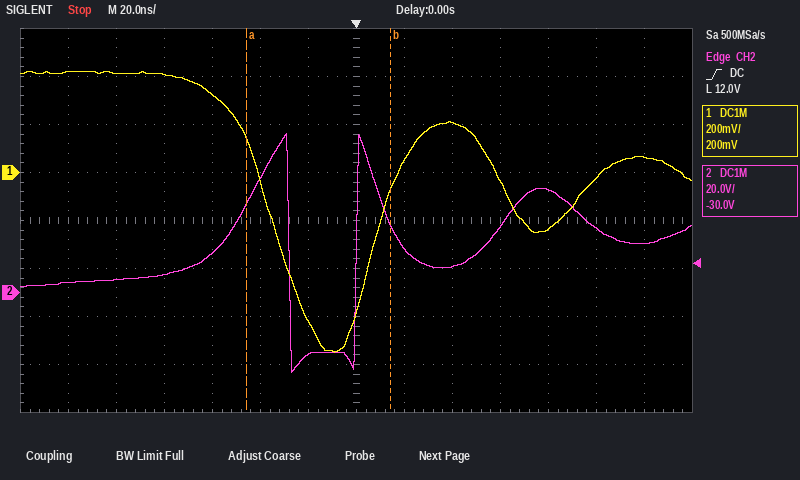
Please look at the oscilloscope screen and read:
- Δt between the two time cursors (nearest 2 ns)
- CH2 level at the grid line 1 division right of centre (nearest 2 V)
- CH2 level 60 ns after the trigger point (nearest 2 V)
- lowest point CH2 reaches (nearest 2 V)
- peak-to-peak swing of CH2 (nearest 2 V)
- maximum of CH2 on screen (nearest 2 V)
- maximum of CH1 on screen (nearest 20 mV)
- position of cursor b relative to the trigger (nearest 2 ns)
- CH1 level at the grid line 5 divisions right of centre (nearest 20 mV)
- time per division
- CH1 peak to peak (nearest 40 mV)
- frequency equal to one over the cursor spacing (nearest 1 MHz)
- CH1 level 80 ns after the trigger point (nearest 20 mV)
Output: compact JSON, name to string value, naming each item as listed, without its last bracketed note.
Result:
{"Δt between the two time cursors": "60 ns", "CH2 level at the grid line 1 division right of centre": "18 V", "CH2 level 60 ns after the trigger point": "28 V", "lowest point CH2 reaches": "-34 V", "peak-to-peak swing of CH2": "100 V", "maximum of CH2 on screen": "66 V", "maximum of CH1 on screen": "420 mV", "position of cursor b relative to the trigger": "+14 ns", "CH1 level at the grid line 5 divisions right of centre": "-20 mV", "time per division": "20 ns", "CH1 peak to peak": "1.16 V", "frequency equal to one over the cursor spacing": "17 MHz", "CH1 level 80 ns after the trigger point": "-240 mV"}
